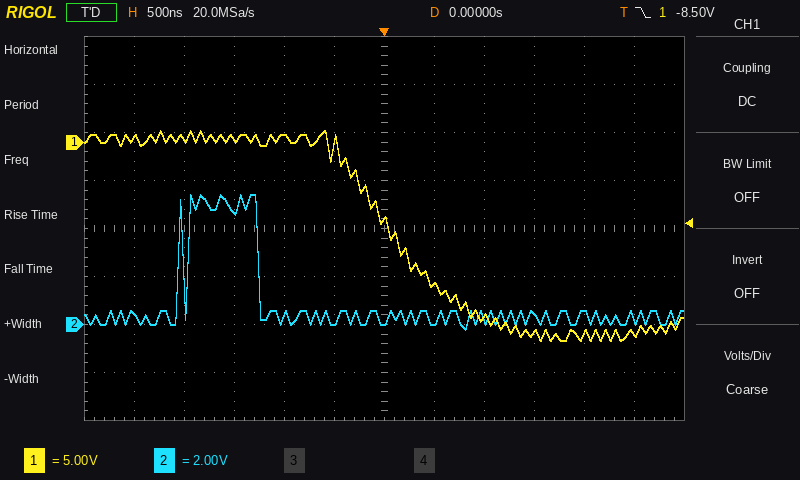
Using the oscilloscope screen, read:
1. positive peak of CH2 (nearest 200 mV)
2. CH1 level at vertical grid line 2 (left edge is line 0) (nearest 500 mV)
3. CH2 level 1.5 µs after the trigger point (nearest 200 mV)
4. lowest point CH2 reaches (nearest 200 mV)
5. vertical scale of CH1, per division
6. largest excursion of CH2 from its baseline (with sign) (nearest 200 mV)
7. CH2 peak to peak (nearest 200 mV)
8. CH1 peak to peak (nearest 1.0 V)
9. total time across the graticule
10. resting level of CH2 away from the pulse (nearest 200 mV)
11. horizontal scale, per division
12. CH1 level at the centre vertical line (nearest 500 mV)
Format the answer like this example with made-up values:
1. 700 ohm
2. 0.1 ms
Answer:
1. 5.4 V
2. 500 mV
3. 400 mV
4. -200 mV
5. 5 V
6. +5.0 V
7. 5.6 V
8. 22.0 V
9. 6 µs
10. 400 mV
11. 500 ns
12. -8.0 V
